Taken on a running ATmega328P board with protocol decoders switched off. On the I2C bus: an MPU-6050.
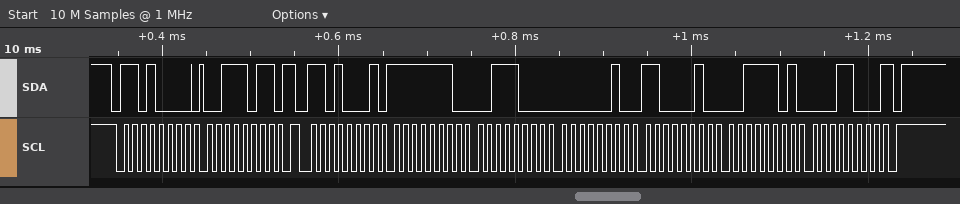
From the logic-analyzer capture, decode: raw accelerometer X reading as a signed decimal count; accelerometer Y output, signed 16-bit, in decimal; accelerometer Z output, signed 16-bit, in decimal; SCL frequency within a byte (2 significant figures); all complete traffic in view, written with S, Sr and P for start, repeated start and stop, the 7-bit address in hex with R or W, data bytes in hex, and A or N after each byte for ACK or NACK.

-456
706
15640
100 kHz
S 68W A 3B A Sr 68R A FE A 38 A 02 A C2 A 3D A 18 N P
